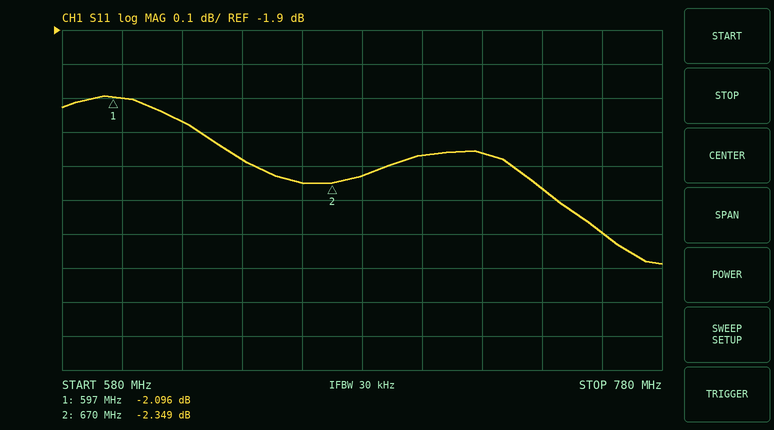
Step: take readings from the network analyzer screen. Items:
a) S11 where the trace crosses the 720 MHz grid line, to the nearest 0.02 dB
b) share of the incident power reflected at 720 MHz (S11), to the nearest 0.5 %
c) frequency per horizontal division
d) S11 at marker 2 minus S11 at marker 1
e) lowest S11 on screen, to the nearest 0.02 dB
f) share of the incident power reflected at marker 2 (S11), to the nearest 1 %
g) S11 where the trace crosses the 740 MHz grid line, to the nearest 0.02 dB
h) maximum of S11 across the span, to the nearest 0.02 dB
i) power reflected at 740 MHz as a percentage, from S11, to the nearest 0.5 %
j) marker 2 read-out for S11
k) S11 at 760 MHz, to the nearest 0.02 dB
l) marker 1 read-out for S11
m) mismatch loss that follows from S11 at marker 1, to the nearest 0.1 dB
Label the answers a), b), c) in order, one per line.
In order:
a) -2.26 dB
b) 59.5 %
c) 20 MHz
d) -0.253 dB
e) -2.58 dB
f) 58 %
g) -2.36 dB
h) -2.10 dB
i) 58.0 %
j) -2.349 dB
k) -2.50 dB
l) -2.096 dB
m) 4.2 dB
